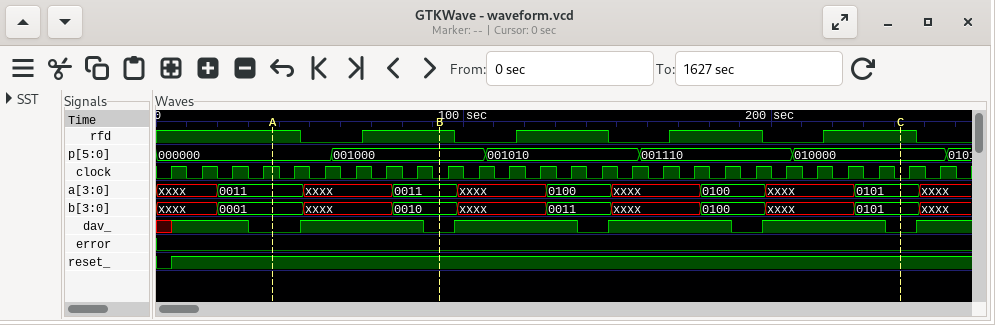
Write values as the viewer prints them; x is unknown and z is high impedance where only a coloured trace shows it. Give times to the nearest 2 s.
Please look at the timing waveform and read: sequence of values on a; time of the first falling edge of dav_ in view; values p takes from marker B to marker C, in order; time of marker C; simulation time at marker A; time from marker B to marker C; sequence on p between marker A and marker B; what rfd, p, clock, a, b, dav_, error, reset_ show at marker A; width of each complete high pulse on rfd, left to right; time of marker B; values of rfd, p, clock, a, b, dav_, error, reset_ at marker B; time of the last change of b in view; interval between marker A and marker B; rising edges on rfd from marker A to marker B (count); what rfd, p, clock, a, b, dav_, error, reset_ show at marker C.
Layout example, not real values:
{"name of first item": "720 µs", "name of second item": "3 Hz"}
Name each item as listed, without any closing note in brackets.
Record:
{"sequence of values on a": "xxxx, 0011, xxxx, 0011, xxxx, 0100, xxxx, 0100, xxxx, 0101, xxxx", "time of the first falling edge of dav_ in view": "30 s", "values p takes from marker B to marker C, in order": "001000, 001010, 001110, 010000", "time of marker C": "242 s", "simulation time at marker A": "38 s", "time from marker B to marker C": "150 s", "sequence on p between marker A and marker B": "000000, 001000", "what rfd, p, clock, a, b, dav_, error, reset_ show at marker A": "rfd=1, p=000000, clock=1, a=0011, b=0001, dav_=0, error=0, reset_=1", "width of each complete high pulse on rfd, left to right": "30 s, 30 s, 30 s, 30 s", "time of marker B": "92 s", "values of rfd, p, clock, a, b, dav_, error, reset_ at marker B": "rfd=1, p=001000, clock=0, a=0011, b=0010, dav_=0, error=0, reset_=1", "time of the last change of b in view": "248 s", "interval between marker A and marker B": "54 s", "rising edges on rfd from marker A to marker B": "1", "what rfd, p, clock, a, b, dav_, error, reset_ show at marker C": "rfd=1, p=010000, clock=0, a=0101, b=0101, dav_=0, error=0, reset_=1"}
